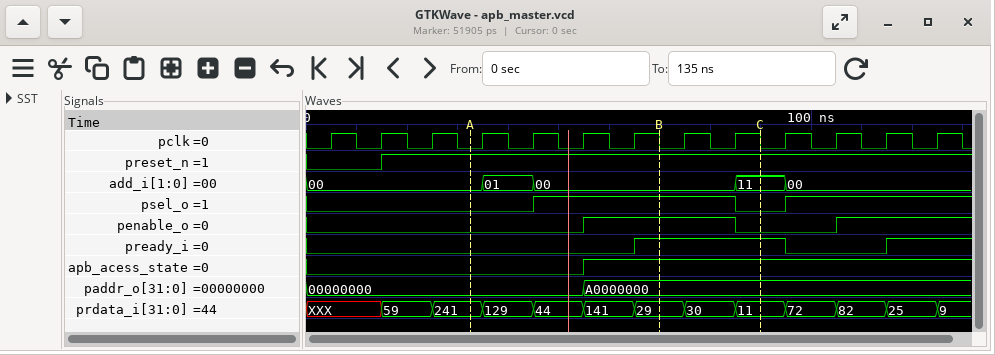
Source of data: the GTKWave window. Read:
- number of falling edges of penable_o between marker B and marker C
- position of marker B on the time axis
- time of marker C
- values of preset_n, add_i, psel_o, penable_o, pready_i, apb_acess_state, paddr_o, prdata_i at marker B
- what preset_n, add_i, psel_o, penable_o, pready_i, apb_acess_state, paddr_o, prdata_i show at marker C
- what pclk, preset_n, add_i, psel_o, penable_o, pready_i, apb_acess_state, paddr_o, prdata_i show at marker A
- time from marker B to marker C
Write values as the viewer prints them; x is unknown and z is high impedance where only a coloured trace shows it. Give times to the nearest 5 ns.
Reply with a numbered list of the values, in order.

1. 1
2. 70 ns
3. 90 ns
4. preset_n=1, add_i=00, psel_o=1, penable_o=1, pready_i=1, apb_acess_state=1, paddr_o=A0000000, prdata_i=29
5. preset_n=1, add_i=11, psel_o=0, penable_o=0, pready_i=1, apb_acess_state=1, paddr_o=A0000000, prdata_i=11
6. pclk=0, preset_n=1, add_i=00, psel_o=0, penable_o=0, pready_i=0, apb_acess_state=0, paddr_o=00000000, prdata_i=241
7. 20 ns
